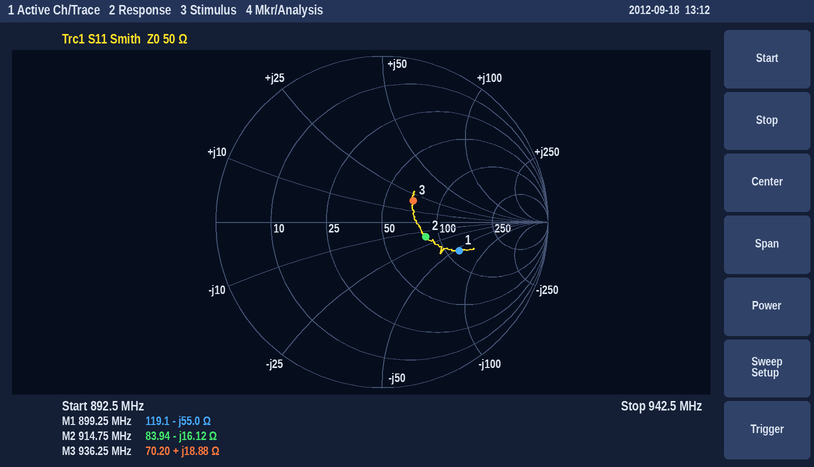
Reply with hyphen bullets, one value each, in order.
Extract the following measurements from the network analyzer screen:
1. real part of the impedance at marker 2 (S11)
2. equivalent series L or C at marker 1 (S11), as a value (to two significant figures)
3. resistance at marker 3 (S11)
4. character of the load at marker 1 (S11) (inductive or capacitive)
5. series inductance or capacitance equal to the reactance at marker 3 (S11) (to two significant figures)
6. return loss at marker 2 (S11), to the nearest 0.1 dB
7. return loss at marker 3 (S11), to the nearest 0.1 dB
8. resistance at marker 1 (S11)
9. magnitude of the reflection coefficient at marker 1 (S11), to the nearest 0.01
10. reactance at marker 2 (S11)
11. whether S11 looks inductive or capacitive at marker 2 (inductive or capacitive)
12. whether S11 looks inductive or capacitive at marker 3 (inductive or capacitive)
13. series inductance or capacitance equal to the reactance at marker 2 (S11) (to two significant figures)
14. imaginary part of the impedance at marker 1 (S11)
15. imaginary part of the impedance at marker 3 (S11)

- 83.94 Ω
- 3.2 pF
- 70.20 Ω
- capacitive
- 3.2 nH
- 11.1 dB
- 12.9 dB
- 119.1 Ω
- 0.50
- -16.12 Ω
- capacitive
- inductive
- 11 pF
- -55.0 Ω
- +18.88 Ω
